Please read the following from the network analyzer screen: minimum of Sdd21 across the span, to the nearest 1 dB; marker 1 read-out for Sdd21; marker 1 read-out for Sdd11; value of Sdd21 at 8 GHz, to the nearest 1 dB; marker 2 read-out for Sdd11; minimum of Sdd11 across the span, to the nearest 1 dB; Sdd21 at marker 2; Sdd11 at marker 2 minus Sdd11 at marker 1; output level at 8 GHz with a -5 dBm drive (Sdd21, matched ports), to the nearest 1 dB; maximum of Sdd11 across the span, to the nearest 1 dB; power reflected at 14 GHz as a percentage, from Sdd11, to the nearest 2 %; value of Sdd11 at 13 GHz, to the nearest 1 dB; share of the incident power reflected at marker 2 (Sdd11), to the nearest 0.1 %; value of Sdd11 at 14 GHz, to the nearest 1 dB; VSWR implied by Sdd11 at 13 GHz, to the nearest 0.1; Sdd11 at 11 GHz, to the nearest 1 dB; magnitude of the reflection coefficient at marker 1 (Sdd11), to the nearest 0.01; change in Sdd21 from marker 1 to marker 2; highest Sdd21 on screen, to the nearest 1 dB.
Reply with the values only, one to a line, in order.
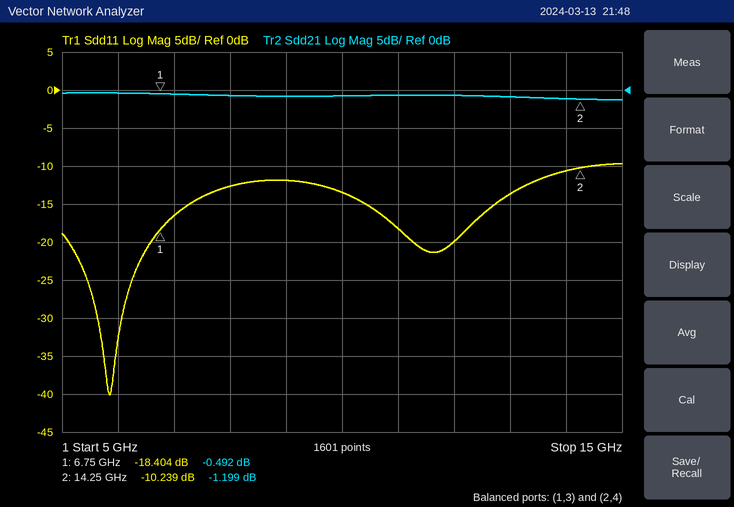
-1 dB
-0.492 dB
-18.404 dB
-1 dB
-10.239 dB
-40 dB
-1.199 dB
8.165 dB
-6 dBm
-10 dB
8 %
-14 dB
9.5 %
-11 dB
1.5
-18 dB
0.12
-0.707 dB
0 dB
